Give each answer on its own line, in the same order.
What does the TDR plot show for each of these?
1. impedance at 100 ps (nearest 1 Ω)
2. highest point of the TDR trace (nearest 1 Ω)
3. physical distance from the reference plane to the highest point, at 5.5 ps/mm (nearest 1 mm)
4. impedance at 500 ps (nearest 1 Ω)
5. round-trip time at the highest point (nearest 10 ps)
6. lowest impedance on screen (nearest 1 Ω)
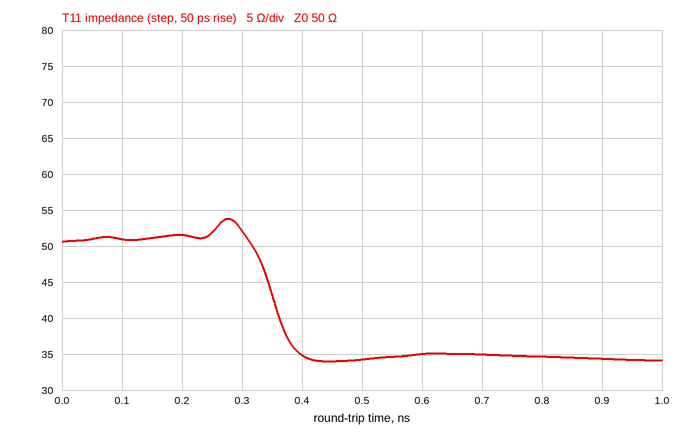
51 Ω
54 Ω
25 mm
34 Ω
280 ps
34 Ω
